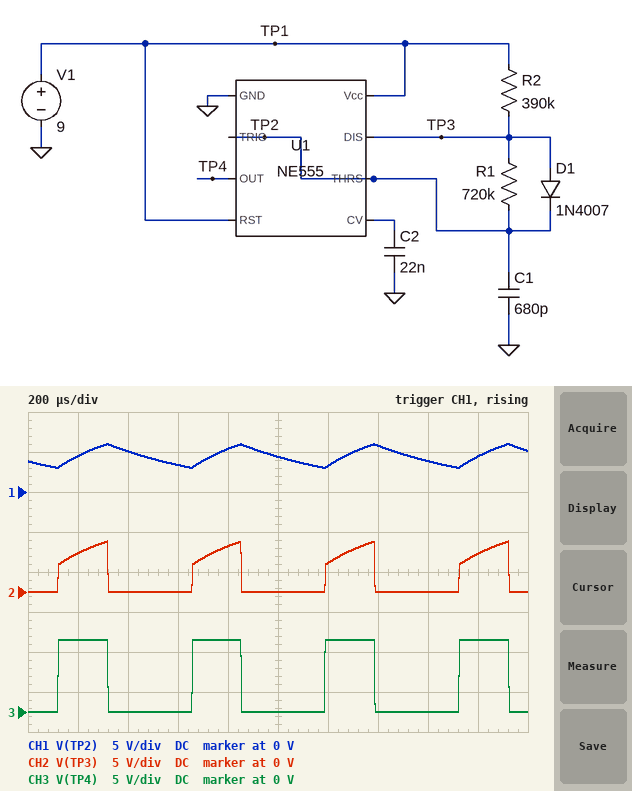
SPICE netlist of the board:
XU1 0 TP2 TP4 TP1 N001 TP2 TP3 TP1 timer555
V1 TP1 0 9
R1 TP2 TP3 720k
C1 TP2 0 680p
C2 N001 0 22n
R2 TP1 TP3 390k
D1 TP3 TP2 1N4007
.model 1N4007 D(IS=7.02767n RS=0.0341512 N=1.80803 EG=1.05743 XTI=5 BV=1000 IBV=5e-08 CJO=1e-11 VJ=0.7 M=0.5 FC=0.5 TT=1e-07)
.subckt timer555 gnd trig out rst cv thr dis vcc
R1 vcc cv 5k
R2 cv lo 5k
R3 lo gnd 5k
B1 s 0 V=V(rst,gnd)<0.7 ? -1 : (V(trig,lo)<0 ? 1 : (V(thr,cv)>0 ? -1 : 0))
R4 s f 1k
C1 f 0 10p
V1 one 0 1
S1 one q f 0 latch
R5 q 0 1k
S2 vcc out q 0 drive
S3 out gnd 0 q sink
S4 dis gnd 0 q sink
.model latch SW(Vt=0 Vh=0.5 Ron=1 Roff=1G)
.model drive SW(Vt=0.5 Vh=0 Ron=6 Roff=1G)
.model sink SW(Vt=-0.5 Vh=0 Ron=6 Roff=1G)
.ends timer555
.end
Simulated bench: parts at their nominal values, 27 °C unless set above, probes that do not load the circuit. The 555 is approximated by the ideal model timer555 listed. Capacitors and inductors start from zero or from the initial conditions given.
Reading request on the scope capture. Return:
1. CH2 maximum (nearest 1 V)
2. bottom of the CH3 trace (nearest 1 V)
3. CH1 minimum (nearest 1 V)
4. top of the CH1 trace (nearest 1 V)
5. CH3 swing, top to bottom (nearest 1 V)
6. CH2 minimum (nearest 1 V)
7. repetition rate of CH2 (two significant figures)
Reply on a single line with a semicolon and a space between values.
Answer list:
6 V; 0 V; 3 V; 6 V; 9 V; 0 V; 1.9 kHz
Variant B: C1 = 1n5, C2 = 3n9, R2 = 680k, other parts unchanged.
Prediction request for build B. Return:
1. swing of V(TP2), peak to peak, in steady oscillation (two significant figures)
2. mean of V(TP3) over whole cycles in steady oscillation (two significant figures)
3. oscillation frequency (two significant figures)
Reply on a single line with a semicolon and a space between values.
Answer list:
3.0 V; 2.5 V; 660 Hz
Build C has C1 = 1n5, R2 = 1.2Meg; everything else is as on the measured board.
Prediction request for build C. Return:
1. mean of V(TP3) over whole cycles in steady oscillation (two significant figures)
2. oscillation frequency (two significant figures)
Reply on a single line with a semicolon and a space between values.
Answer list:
3.2 V; 480 Hz
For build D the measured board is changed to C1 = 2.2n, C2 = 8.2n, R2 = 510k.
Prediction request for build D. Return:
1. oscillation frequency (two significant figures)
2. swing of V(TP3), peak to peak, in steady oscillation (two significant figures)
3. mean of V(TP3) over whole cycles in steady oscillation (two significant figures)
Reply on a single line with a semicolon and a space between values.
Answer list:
520 Hz; 6.3 V; 2.2 V
